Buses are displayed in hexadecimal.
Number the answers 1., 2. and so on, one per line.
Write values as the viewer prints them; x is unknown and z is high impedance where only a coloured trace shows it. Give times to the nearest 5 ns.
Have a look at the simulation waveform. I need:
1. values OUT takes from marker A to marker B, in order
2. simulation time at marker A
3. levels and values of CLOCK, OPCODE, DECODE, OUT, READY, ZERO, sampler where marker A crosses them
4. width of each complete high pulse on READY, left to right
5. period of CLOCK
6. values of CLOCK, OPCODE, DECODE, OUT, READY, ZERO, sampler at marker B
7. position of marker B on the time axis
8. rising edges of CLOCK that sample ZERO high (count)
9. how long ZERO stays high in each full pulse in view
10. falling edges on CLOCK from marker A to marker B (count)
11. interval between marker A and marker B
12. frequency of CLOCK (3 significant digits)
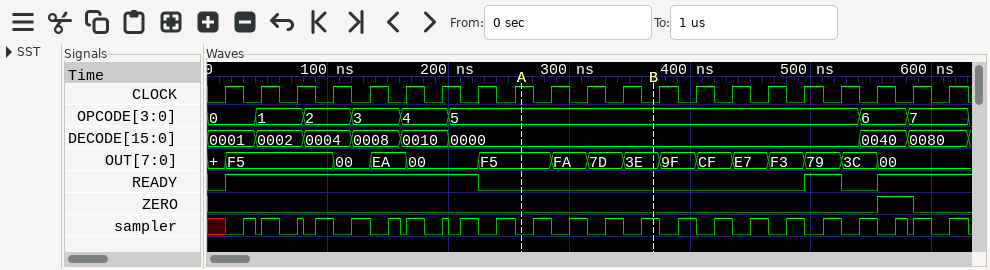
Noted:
1. F5, FA, 7D, 3E
2. 260 ns
3. CLOCK=1, OPCODE=5, DECODE=0000, OUT=F5, READY=0, ZERO=0, sampler=0
4. 210 ns, 30 ns
5. 30 ns
6. CLOCK=0, OPCODE=5, DECODE=0000, OUT=3E, READY=0, ZERO=0, sampler=1
7. 370 ns
8. 1
9. 30 ns
10. 4
11. 110 ns
12. 33.3 MHz
